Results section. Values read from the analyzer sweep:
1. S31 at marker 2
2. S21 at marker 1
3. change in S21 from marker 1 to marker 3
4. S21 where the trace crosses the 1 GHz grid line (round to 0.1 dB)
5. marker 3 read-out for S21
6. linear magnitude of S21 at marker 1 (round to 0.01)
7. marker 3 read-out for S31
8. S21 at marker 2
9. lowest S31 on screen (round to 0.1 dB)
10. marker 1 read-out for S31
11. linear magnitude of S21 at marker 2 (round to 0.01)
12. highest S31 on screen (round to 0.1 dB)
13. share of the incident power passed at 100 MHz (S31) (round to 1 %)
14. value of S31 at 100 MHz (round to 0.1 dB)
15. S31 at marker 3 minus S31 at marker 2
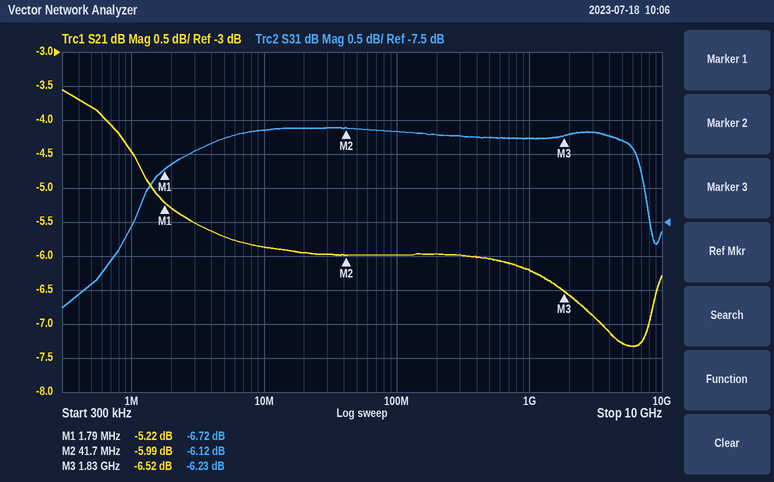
-6.12 dB
-5.22 dB
-1.30 dB
-6.2 dB
-6.52 dB
0.55
-6.23 dB
-5.99 dB
-8.8 dB
-6.72 dB
0.50
-6.1 dB
24 %
-6.2 dB
-0.11 dB
